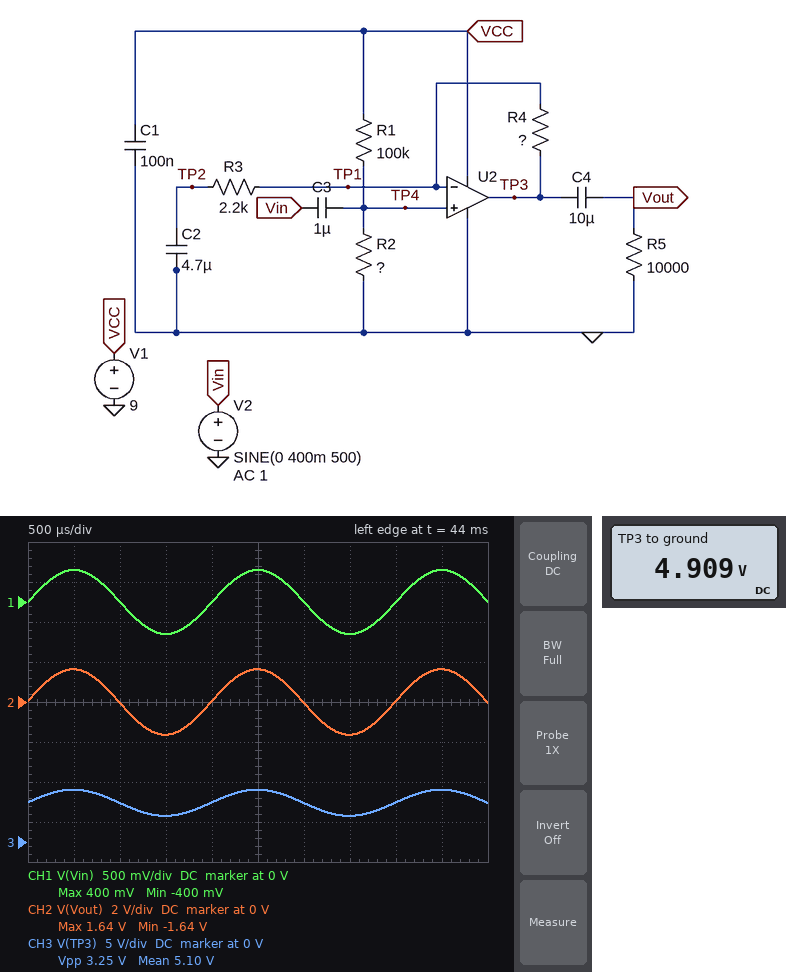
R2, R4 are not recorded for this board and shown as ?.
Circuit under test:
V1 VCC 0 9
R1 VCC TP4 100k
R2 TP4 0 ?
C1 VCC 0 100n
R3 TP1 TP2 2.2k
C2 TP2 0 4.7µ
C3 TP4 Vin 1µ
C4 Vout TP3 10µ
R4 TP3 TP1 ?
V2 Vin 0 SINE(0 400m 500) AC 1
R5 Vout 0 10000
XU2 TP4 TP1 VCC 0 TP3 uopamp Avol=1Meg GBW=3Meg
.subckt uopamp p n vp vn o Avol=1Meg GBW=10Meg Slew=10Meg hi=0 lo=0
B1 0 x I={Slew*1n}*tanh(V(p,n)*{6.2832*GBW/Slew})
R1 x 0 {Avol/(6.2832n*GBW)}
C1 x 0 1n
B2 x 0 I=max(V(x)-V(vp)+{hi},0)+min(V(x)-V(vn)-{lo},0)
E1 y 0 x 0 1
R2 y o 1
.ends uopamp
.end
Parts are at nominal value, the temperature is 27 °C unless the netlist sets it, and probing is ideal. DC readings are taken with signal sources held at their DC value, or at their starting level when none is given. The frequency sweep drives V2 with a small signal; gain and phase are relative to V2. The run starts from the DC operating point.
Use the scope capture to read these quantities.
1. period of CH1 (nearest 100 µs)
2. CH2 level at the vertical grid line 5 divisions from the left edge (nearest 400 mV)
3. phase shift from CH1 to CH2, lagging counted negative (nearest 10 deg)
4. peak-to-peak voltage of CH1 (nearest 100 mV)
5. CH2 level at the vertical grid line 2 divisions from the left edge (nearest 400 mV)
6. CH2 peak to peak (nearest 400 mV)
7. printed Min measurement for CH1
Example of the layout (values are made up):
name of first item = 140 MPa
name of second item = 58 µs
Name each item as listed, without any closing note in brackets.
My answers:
period of CH1 = 2.0 ms
CH2 level at the vertical grid line 5 divisions from the left edge = 1.6 V
phase shift from CH1 to CH2, lagging counted negative = 0 deg
peak-to-peak voltage of CH1 = 800 mV
CH2 level at the vertical grid line 2 divisions from the left edge = 0 V
CH2 peak to peak = 3.2 V
printed Min measurement for CH1 = -400 mV
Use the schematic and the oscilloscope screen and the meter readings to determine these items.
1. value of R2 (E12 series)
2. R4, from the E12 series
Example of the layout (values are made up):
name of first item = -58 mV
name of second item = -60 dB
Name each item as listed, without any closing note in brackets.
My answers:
value of R2 = 120 kΩ
R4, from the E12 series = 6.8 kΩ
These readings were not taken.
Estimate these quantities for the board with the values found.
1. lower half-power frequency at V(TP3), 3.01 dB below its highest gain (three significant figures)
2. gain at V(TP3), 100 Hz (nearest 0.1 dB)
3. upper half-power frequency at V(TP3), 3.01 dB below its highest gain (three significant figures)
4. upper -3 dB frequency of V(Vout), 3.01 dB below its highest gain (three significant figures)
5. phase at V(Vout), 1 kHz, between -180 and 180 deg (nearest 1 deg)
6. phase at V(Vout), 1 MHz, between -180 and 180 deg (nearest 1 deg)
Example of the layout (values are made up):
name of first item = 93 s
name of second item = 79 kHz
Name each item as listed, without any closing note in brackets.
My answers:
lower half-power frequency at V(TP3), 3.01 dB below its highest gain = 15.0 Hz
gain at V(TP3), 100 Hz = 12.1 dB
upper half-power frequency at V(TP3), 3.01 dB below its highest gain = 733 kHz
upper -3 dB frequency of V(Vout), 3.01 dB below its highest gain = 733 kHz
phase at V(Vout), 1 kHz, between -180 and 180 deg = 1 deg
phase at V(Vout), 1 MHz, between -180 and 180 deg = -54 deg
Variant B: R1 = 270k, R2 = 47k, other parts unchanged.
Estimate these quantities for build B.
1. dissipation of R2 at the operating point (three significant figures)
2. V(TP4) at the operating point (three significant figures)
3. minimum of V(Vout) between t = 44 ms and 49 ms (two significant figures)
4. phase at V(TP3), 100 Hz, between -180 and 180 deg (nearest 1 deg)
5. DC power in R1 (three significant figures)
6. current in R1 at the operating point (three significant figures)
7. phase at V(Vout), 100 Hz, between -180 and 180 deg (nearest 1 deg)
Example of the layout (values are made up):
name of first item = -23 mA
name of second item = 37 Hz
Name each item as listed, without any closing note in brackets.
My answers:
dissipation of R2 at the operating point = 37.9 µW
V(TP4) at the operating point = 1.33 V
minimum of V(Vout) between t = 44 ms and 49 ms = -1.3 V
phase at V(TP3), 100 Hz, between -180 and 180 deg = 9 deg
DC power in R1 = 218 µW
current in R1 at the operating point = 28.4 µA
phase at V(Vout), 100 Hz, between -180 and 180 deg = 10 deg
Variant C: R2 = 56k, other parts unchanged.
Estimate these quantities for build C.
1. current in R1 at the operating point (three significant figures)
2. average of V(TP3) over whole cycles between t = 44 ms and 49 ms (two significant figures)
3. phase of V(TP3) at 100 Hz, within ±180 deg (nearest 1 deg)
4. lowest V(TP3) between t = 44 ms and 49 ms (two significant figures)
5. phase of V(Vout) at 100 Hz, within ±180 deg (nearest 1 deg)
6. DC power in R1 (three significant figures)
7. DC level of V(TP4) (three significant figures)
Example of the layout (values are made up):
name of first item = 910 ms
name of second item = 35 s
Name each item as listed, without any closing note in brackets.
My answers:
current in R1 at the operating point = 57.7 µA
average of V(TP3) over whole cycles between t = 44 ms and 49 ms = 3.2 V
phase of V(TP3) at 100 Hz, within ±180 deg = 9 deg
lowest V(TP3) between t = 44 ms and 49 ms = 1.6 V
phase of V(Vout) at 100 Hz, within ±180 deg = 10 deg
DC power in R1 = 333 µW
DC level of V(TP4) = 3.23 V
